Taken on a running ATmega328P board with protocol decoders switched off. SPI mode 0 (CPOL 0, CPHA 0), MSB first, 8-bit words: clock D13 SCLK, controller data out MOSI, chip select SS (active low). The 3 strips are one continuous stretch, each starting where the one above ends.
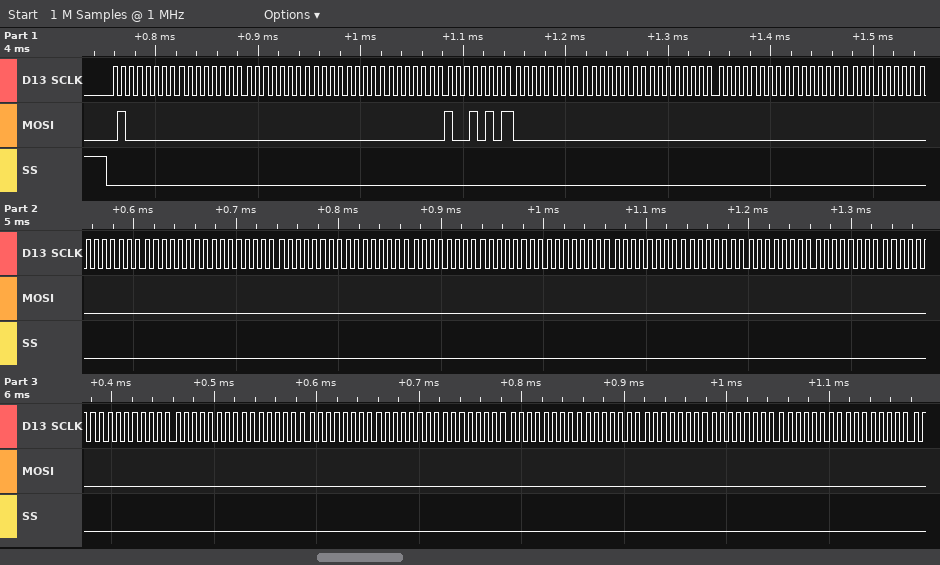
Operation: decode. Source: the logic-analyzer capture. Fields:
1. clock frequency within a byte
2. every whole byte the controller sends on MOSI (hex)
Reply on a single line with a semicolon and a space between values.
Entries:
125 kHz; 40 00 00 00 00 95 00 00 00 00 00 00 00 00 00 00 00 00 00 00 00 00 00 00 00 00 00 00 00 00 00 00 00 00 00 00 00
